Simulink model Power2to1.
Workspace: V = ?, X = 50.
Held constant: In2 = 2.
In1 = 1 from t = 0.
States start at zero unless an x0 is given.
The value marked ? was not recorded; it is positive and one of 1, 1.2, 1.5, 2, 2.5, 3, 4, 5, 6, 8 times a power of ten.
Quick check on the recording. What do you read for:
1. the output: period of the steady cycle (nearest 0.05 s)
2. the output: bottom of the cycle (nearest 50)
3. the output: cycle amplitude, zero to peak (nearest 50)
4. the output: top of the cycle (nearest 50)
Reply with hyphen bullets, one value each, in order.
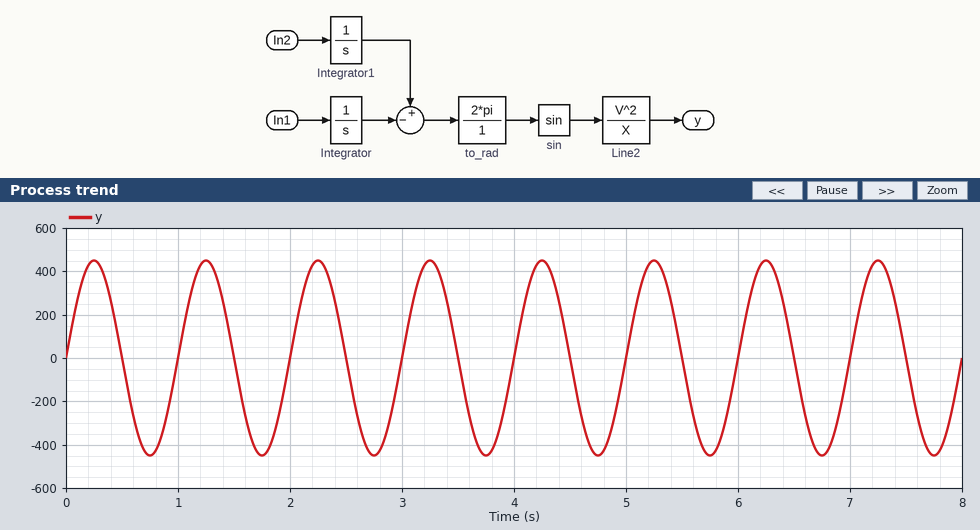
- 1.00 s
- -450
- 450
- 450
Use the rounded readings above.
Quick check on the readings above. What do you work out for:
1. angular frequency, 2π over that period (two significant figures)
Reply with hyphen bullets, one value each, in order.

- 6.3 rad/s
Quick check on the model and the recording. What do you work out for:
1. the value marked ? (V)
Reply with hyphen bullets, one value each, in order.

- 150
